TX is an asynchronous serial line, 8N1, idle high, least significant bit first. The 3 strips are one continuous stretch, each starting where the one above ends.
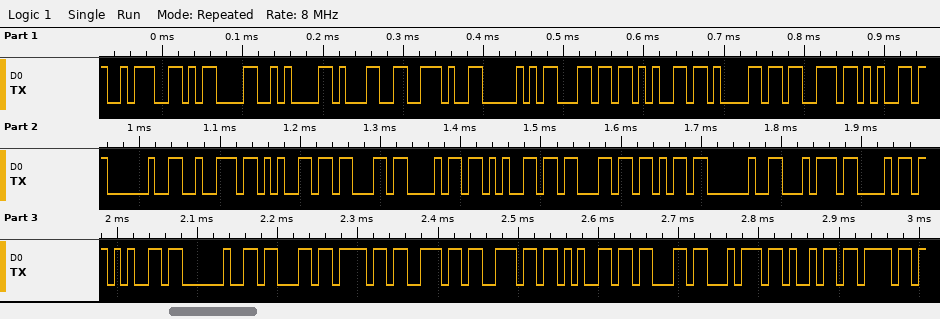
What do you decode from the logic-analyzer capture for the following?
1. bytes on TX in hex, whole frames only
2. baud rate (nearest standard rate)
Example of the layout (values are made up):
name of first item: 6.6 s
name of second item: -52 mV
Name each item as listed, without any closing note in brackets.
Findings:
bytes on TX in hex, whole frames only: 3A 0D 0A 31 2E 50 6C 65 61 73 65 20 72 65 63 68 65 63 6B 20 74 68 65 20 63 6F 6E 6E 65 63 74 69 6F
baud rate: 115200 baud
